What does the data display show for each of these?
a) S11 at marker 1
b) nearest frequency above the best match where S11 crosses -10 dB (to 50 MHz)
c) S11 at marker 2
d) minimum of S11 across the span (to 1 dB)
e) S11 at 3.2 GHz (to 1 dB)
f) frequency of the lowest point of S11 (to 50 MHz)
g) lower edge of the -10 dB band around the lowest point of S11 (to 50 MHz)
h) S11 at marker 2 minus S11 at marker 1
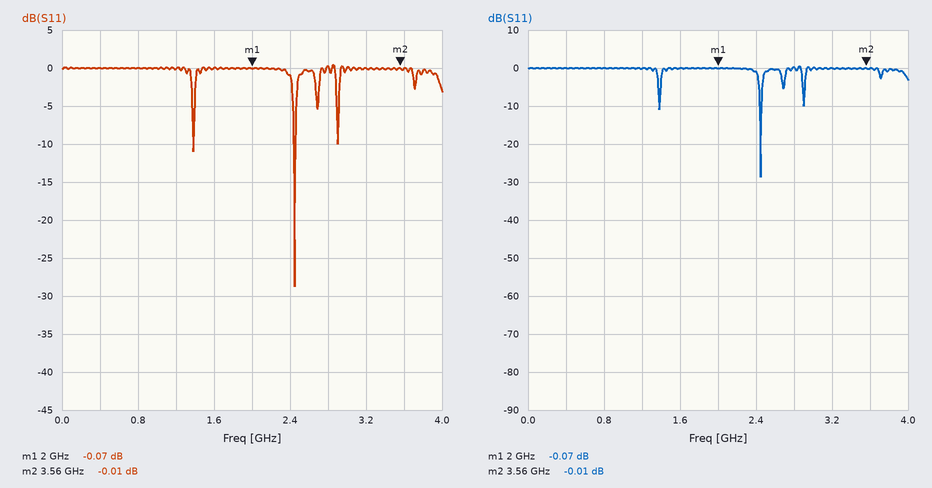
-0.07 dB
2.45 GHz
-0.01 dB
-29 dB
0 dB
2.45 GHz
2.45 GHz
0.06 dB
